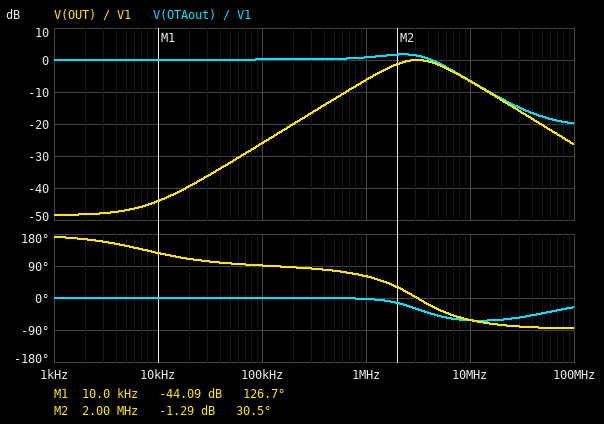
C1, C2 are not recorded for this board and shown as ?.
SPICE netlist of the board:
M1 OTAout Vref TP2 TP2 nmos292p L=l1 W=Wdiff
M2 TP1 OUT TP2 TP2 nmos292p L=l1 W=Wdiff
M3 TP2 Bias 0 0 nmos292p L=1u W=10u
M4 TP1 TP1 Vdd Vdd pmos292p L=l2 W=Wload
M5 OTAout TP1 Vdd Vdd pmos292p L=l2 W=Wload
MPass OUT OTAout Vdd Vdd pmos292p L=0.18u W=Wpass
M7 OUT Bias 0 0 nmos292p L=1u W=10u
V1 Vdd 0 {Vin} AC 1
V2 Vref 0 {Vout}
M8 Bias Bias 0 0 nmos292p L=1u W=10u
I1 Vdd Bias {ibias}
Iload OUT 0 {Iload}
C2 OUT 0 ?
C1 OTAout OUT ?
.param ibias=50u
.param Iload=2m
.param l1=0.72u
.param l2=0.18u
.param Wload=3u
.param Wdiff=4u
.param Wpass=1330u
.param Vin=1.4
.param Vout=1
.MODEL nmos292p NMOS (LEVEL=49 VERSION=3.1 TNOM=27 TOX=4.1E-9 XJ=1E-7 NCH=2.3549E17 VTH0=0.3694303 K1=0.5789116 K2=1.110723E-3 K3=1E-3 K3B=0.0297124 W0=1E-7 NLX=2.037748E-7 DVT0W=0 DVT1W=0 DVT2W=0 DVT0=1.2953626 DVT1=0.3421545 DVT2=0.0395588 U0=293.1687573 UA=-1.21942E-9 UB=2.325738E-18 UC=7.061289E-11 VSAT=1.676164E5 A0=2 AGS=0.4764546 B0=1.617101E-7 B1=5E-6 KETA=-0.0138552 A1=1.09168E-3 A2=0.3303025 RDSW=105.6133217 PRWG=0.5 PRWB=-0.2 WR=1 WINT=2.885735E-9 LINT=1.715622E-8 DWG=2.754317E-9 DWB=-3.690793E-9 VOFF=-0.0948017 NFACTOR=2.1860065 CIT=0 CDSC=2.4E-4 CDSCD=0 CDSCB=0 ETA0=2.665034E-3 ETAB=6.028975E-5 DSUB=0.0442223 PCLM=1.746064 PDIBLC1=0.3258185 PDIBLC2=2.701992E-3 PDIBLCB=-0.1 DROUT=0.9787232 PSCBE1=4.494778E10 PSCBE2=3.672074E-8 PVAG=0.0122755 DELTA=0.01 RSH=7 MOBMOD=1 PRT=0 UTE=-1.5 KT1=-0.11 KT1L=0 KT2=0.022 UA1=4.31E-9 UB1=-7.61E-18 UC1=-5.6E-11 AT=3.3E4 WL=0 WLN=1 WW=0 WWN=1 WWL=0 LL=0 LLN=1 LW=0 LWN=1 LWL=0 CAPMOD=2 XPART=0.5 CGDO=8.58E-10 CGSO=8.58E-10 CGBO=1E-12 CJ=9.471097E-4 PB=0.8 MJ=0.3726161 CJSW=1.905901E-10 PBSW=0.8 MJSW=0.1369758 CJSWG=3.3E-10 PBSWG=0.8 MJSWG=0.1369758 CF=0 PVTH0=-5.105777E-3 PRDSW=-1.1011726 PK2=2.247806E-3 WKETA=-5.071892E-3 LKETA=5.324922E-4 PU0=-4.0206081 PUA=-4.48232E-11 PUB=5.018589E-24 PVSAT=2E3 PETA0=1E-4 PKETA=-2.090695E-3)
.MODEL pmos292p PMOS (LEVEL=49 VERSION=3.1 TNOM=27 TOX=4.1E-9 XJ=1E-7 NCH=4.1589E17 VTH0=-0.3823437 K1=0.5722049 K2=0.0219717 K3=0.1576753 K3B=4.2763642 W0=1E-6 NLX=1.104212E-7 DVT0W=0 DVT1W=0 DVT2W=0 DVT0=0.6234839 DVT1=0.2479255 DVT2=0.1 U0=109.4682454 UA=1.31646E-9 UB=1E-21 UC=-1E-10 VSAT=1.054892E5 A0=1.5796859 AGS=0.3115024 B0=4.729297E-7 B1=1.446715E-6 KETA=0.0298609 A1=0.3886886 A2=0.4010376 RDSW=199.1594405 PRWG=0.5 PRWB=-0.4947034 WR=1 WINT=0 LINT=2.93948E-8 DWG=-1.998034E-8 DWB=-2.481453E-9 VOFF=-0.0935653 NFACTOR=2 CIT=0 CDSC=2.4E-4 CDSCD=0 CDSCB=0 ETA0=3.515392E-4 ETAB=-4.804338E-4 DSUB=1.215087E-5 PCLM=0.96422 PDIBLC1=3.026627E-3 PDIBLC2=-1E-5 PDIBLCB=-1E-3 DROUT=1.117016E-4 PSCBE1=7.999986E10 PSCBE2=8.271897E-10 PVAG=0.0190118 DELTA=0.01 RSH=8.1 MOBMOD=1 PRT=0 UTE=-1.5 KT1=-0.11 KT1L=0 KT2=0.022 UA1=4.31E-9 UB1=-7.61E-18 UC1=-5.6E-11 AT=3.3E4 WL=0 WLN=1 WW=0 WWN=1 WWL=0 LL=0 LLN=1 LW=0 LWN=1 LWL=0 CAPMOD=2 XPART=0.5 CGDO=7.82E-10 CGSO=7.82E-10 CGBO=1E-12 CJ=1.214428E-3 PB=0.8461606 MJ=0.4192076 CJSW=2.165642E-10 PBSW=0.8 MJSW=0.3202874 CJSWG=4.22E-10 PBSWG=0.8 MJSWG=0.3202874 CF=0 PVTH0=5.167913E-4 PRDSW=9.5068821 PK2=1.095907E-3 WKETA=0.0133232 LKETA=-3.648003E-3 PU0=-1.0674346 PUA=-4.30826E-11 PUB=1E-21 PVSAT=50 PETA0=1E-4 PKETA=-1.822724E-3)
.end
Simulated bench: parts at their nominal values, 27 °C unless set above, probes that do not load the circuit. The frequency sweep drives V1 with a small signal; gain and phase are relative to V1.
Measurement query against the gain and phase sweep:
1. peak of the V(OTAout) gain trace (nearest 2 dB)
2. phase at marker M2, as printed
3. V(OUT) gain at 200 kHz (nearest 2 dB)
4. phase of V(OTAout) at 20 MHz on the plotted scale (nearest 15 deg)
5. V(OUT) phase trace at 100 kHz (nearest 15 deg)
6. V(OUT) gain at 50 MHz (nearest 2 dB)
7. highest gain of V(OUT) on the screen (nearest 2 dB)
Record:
2 dB
30.5 deg
-20 dB
-60 deg
90 deg
-20 dB
0 dB
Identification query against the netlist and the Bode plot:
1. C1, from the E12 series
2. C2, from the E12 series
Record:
18 pF
820 pF
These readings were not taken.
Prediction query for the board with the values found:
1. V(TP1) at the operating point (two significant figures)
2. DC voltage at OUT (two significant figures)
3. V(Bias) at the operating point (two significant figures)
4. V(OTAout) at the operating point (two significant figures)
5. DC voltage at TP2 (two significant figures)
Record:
750 mV
1.0 V
620 mV
840 mV
380 mV
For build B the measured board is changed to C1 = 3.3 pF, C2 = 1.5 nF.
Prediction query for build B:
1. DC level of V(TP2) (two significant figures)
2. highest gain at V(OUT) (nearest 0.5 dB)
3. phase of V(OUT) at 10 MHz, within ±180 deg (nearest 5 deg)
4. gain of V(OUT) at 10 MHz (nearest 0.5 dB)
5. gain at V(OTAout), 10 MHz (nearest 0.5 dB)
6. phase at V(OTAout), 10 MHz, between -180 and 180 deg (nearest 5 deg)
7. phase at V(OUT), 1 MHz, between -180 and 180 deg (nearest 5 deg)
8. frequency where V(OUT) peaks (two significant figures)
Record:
380 mV
-0.5 dB
-75 deg
-12.5 dB
-10.5 dB
-45 deg
85 deg
4.2 MHz
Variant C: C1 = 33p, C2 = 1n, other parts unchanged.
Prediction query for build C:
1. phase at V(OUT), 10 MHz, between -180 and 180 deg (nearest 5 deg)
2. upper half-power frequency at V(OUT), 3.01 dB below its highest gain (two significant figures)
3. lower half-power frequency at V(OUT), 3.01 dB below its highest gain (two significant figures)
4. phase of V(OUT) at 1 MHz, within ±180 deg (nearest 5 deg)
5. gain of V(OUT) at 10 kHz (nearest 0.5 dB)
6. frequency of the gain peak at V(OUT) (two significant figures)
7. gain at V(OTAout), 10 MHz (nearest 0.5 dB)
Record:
-65 deg
5.0 MHz
920 kHz
40 deg
-40.5 dB
2.1 MHz
-8.0 dB
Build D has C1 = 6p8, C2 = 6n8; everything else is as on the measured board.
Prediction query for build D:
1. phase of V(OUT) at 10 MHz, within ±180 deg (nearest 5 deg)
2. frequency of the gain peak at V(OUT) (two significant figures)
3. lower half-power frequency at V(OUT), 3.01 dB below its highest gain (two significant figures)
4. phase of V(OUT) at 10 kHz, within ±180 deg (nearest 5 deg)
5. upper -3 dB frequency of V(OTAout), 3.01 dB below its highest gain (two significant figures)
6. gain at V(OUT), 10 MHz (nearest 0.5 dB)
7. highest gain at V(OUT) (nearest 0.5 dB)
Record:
-85 deg
1.6 MHz
1.3 MHz
150 deg
1.8 MHz
-25.5 dB
-2.0 dB
